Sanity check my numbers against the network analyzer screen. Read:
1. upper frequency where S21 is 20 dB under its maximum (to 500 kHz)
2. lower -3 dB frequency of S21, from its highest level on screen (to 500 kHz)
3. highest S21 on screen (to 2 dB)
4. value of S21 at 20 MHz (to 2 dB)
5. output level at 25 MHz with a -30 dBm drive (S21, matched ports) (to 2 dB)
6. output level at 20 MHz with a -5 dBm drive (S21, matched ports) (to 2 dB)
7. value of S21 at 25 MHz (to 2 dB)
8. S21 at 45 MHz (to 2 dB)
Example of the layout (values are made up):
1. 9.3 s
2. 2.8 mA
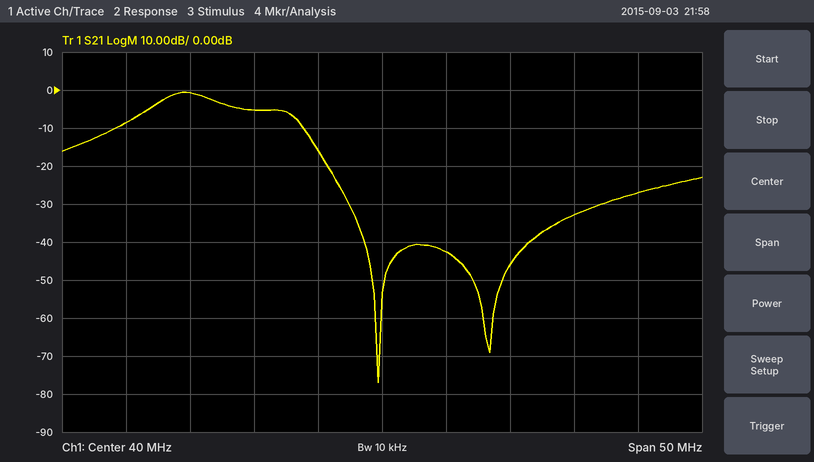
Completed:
1. 36.0 MHz
2. 22.5 MHz
3. 0 dB
4. -8 dB
5. -30 dBm
6. -14 dBm
7. 0 dB
8. -42 dB
